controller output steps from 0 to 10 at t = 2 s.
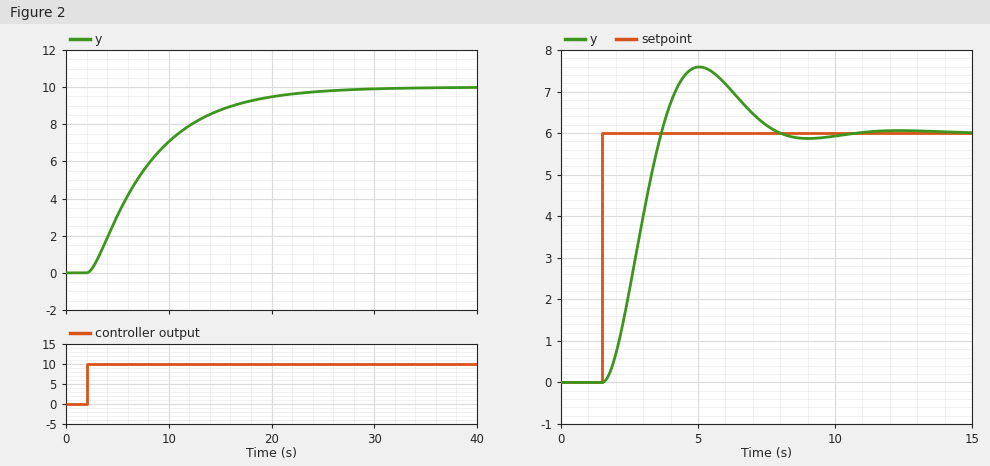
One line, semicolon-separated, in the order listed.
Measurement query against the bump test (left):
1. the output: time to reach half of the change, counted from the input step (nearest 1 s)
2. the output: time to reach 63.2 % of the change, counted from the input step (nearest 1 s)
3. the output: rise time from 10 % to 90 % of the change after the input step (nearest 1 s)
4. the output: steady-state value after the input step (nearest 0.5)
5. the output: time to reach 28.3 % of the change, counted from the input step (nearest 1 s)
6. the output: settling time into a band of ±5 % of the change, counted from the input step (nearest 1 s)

5 s; 7 s; 13 s; 10.0; 3 s; 18 s
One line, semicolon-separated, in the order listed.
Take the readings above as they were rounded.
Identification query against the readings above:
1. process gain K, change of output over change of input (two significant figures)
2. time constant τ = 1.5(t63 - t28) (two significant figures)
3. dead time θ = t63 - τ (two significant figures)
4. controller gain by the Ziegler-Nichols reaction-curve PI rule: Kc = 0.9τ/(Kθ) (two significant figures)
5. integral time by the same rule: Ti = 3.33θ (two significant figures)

1.0; 6.0 s; 1.0 s; 5.4; 3.3 s
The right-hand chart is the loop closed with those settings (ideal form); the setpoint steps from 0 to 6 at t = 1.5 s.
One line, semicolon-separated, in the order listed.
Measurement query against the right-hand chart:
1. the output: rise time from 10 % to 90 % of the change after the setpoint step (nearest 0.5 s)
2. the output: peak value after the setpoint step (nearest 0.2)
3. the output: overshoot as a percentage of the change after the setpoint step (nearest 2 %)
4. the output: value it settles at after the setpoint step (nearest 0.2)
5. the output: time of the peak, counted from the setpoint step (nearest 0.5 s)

1.5 s; 7.6; 26 %; 6.0; 3.5 s
